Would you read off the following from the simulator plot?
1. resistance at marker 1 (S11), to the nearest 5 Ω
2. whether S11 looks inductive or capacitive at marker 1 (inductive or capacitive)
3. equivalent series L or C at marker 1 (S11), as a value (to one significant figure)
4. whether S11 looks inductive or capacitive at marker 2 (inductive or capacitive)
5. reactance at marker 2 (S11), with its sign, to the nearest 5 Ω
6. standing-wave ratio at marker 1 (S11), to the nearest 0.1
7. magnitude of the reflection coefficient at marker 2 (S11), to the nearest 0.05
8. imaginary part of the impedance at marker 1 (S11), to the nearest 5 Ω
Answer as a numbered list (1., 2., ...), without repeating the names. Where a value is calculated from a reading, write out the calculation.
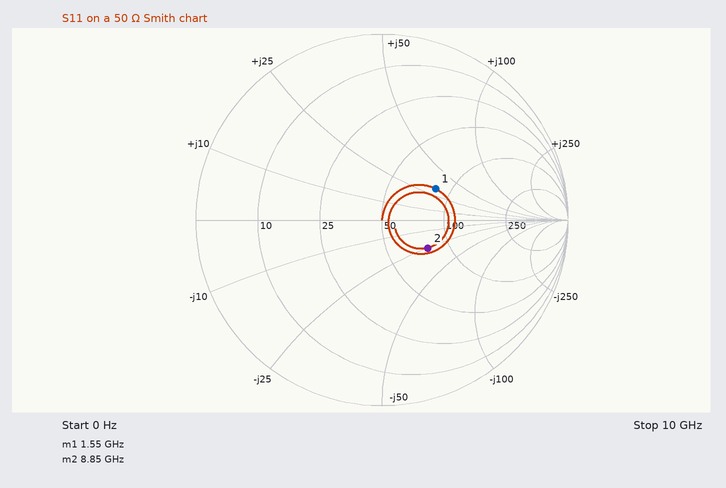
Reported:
1. 85 Ω
2. inductive
3. L = 30 Ω/(2π × 1.55 GHz) ≈ 3 nH
4. capacitive
5. -25 Ω
6. 2.0
7. 0.30
8. +30 Ω
